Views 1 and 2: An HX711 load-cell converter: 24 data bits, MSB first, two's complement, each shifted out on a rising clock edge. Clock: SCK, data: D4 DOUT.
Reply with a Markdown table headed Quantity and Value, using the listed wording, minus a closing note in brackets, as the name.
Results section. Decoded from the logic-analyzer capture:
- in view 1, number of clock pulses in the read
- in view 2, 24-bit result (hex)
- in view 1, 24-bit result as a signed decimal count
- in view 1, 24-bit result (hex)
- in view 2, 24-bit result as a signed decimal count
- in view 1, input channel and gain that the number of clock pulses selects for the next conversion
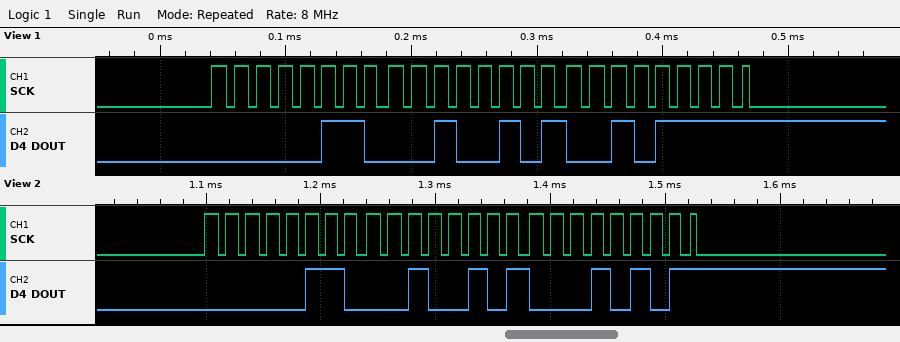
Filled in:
| Quantity | Value |
|---|---|
| in view 1, number of clock pulses in the read | 25 |
| in view 2, 24-bit result | 0x062515 |
| in view 1, 24-bit result as a signed decimal count | 402735 |
| in view 1, 24-bit result | 0x06252F |
| in view 2, 24-bit result as a signed decimal count | 402709 |
| in view 1, input channel and gain that the number of clock pulses selects for the next conversion | channel A, gain 128 |
